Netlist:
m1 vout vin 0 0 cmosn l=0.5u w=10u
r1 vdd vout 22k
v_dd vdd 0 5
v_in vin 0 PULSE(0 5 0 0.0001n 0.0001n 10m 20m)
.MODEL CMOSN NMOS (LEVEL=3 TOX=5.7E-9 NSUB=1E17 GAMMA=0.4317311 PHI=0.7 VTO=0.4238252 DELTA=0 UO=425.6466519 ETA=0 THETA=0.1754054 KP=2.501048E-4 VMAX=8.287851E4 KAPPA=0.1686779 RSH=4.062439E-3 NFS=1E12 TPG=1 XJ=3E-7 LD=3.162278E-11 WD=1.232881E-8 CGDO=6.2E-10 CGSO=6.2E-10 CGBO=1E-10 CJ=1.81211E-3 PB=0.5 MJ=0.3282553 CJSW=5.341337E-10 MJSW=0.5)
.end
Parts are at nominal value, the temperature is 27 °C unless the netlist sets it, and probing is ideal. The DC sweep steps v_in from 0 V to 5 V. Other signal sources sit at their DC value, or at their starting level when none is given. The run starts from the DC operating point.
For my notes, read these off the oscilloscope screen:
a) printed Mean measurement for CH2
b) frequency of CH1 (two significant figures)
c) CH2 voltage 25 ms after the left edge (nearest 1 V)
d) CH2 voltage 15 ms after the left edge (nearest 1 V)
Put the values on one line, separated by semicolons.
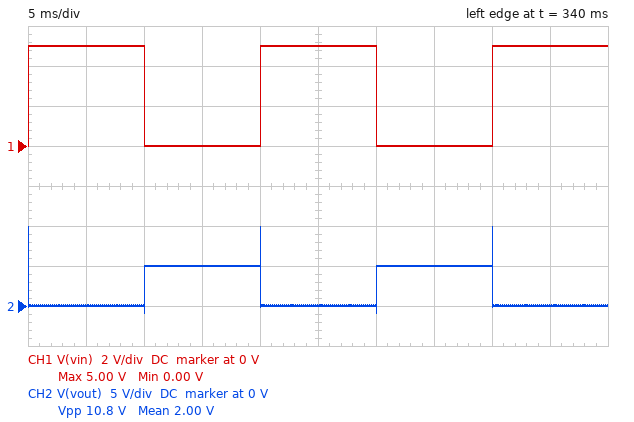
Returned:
2.00 V; 50 Hz; 0 V; 5 V
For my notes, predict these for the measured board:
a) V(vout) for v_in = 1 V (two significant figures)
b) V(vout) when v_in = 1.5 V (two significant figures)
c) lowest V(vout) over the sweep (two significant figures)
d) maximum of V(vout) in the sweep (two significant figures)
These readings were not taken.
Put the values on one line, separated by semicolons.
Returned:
91 mV; 51 mV; 18 mV; 5.0 V
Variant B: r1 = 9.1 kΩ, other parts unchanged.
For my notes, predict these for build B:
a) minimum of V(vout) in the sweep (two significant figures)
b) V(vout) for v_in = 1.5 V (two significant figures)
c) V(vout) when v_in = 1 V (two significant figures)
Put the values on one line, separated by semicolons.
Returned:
44 mV; 130 mV; 320 mV
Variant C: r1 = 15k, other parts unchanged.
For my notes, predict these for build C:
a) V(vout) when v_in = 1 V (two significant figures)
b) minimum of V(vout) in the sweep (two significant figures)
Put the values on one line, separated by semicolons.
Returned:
150 mV; 26 mV
